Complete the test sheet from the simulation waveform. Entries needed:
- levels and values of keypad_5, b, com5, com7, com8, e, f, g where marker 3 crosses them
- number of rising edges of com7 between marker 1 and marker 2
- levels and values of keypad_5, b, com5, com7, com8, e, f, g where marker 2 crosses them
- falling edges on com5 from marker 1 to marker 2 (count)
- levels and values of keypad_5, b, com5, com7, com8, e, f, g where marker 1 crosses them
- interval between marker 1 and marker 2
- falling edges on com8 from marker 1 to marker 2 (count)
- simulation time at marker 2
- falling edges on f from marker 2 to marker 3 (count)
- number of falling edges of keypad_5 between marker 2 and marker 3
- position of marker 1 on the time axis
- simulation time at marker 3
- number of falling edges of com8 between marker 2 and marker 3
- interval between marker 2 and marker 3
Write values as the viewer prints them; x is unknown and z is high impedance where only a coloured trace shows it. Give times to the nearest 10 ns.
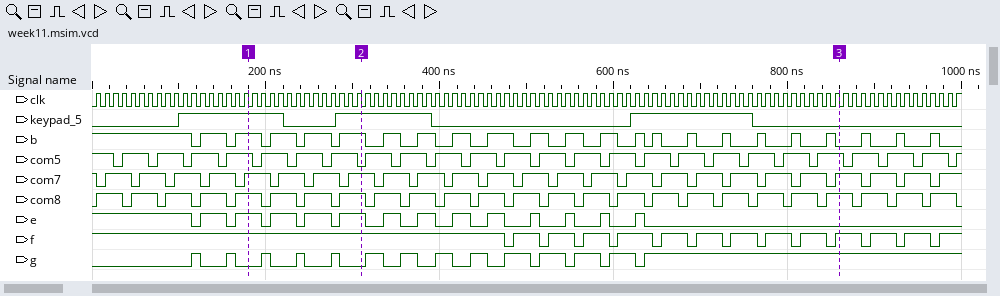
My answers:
keypad_5=0, b=0, com5=1, com7=1, com8=1, e=0, f=1, g=1
3
keypad_5=1, b=1, com5=0, com7=1, com8=1, e=1, f=1, g=0
4
keypad_5=1, b=1, com5=1, com7=1, com8=1, e=1, f=1, g=0
130 ns
3
310 ns
10
2
180 ns
860 ns
14
550 ns
